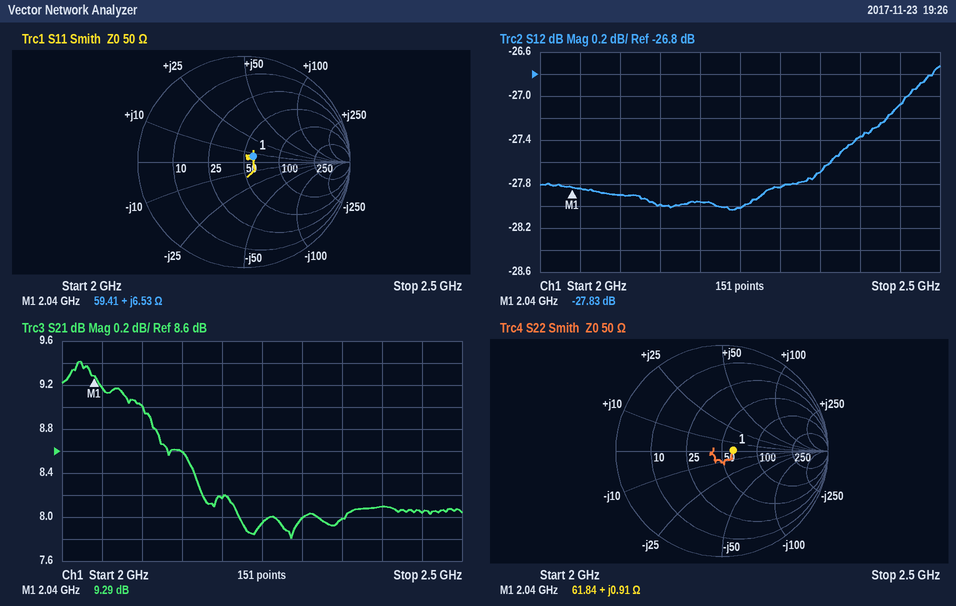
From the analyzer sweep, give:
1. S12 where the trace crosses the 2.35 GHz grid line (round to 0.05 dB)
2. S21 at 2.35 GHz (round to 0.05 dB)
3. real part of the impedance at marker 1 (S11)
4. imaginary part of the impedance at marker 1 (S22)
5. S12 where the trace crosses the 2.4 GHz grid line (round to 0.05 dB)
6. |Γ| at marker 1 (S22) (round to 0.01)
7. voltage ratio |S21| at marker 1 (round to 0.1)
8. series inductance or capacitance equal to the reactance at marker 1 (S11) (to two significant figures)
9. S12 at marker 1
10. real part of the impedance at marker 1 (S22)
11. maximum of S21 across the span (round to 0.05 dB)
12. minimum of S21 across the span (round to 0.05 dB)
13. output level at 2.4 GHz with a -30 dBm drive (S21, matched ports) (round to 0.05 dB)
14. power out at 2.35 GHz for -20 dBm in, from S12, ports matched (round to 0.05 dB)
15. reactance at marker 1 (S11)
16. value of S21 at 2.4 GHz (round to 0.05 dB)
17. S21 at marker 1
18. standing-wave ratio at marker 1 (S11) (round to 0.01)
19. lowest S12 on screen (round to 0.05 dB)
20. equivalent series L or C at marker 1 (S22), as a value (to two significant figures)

-27.70 dB
8.00 dB
59.41 Ω
+0.91 Ω
-27.35 dB
0.11
2.9
510 pH
-27.83 dB
61.84 Ω
9.40 dB
7.80 dB
-21.90 dBm
-47.70 dBm
+6.53 Ω
8.10 dB
9.29 dB
1.23
-28.05 dB
71 pH
